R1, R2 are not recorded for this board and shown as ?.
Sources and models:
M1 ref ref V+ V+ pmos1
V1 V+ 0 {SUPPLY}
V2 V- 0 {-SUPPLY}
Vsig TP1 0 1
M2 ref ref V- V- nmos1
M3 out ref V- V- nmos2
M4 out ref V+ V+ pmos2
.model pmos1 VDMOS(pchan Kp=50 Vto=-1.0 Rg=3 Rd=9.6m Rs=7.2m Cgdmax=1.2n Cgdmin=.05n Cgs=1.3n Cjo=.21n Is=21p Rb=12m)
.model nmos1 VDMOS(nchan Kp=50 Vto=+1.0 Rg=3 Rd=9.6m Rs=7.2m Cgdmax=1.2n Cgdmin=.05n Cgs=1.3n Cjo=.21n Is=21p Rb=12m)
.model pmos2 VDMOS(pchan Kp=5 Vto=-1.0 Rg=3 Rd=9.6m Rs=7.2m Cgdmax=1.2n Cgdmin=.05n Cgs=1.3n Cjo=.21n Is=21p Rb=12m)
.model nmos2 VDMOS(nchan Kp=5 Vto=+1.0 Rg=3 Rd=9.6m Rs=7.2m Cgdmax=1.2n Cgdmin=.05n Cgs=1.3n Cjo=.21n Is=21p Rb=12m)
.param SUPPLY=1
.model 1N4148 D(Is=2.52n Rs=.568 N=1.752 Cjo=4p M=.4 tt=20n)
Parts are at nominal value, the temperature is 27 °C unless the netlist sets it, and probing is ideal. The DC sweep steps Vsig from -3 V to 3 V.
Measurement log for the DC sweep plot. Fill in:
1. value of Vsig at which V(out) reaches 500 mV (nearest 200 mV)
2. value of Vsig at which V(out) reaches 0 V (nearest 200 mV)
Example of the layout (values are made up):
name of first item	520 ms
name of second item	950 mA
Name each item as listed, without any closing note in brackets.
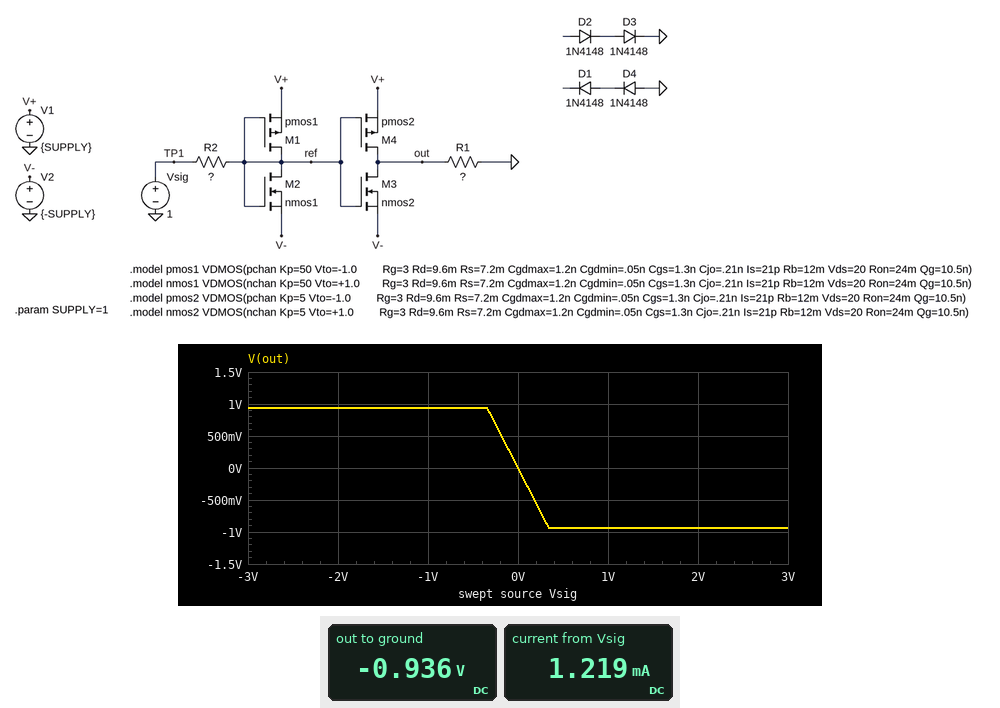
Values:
value of Vsig at which V(out) reaches 500 mV	-200 mV
value of Vsig at which V(out) reaches 0 V	0 V
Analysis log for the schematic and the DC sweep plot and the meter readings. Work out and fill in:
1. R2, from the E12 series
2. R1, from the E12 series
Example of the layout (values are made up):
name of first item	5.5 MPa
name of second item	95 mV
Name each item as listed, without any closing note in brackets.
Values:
R2, from the E12 series	820 Ω
R1, from the E12 series	22 kΩ
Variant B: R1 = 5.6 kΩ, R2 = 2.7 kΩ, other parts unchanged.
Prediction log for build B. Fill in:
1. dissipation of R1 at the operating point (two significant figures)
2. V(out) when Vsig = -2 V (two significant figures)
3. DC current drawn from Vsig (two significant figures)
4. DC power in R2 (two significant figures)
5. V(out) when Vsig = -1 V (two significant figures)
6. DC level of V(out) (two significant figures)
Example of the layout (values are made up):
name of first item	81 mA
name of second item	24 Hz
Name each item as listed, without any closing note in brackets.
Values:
dissipation of R1 at the operating point	8.0 µW
V(out) when Vsig = -2 V	420 mV
DC current drawn from Vsig	370 µA
DC power in R2	370 µW
V(out) when Vsig = -1 V	210 mV
DC level of V(out)	-210 mV
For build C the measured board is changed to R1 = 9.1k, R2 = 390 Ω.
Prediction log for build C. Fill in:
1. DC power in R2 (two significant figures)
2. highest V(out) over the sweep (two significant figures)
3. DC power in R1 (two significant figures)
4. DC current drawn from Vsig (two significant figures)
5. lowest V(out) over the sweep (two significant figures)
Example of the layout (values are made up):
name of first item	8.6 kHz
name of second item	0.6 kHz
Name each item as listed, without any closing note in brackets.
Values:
DC power in R2	2.6 mW
highest V(out) over the sweep	950 mV
DC power in R1	97 µW
DC current drawn from Vsig	2.6 mA
lowest V(out) over the sweep	-950 mV
